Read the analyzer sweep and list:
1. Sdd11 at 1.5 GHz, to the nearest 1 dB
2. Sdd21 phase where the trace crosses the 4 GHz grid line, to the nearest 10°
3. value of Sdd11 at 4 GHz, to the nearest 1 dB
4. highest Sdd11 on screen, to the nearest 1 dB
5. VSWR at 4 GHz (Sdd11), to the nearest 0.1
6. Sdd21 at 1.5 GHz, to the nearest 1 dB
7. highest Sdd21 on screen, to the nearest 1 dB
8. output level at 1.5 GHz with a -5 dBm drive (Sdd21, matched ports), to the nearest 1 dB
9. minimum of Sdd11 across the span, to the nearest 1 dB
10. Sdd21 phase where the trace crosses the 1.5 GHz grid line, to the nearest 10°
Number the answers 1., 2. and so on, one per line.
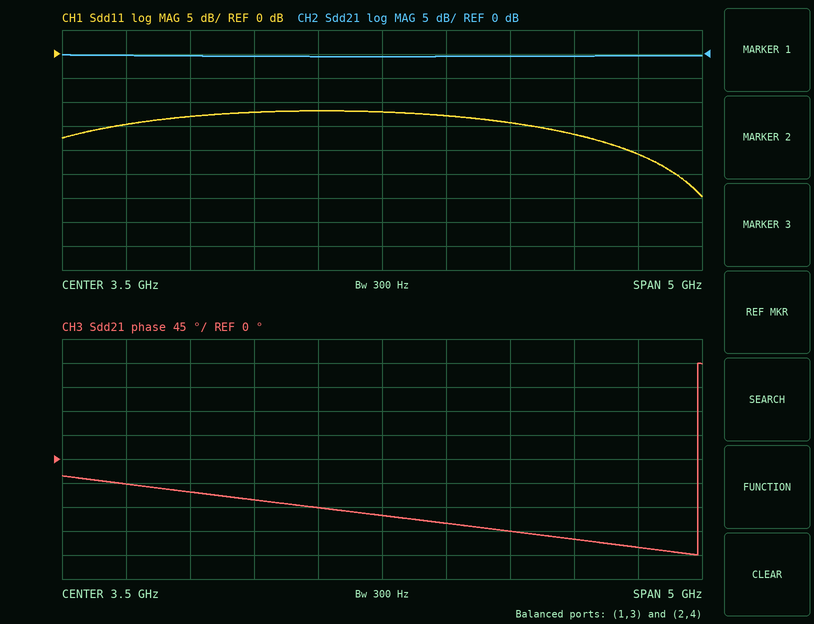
1. -15 dB
2. -120°
3. -13 dB
4. -12 dB
5. 1.6
6. 0 dB
7. 0 dB
8. -5 dBm
9. -30 dB
10. -50°
